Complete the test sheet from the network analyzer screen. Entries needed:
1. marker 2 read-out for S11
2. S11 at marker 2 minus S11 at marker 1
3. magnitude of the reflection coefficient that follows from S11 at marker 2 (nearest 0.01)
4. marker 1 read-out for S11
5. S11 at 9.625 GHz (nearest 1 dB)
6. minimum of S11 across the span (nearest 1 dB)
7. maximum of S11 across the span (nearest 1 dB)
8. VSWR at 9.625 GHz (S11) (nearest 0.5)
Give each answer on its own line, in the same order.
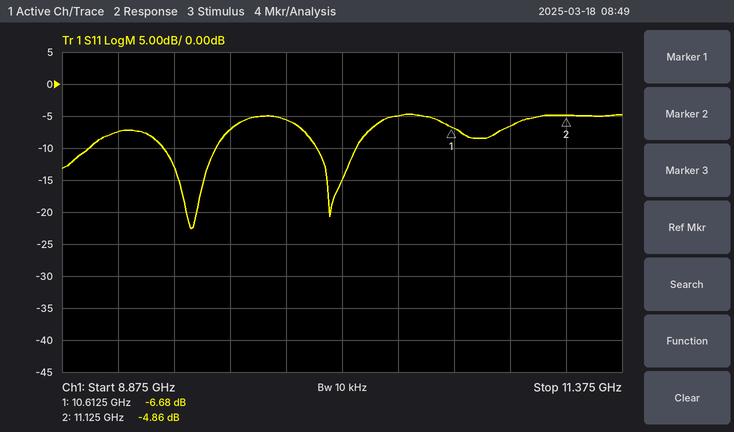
-4.86 dB
1.82 dB
0.57
-6.68 dB
-7 dB
-23 dB
-5 dB
2.5
